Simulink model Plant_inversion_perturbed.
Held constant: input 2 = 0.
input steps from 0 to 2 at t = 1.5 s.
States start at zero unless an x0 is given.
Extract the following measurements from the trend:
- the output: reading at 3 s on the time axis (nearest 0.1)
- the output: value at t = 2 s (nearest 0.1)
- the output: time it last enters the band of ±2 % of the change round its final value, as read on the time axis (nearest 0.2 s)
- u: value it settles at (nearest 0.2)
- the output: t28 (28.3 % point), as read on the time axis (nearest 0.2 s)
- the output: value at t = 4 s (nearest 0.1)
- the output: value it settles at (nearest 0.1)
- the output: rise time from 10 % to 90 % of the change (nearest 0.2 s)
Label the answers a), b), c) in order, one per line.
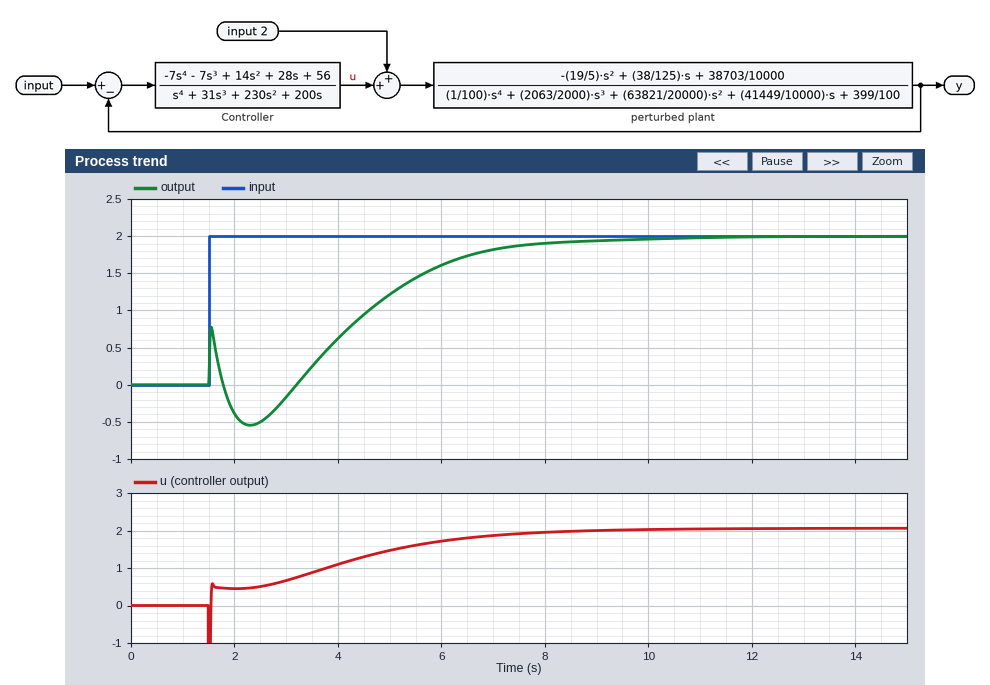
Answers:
a) -0.2
b) -0.4
c) 10.0 s
d) 2.0
e) 1.6 s
f) 0.6
g) 2.0
h) 5.4 s
